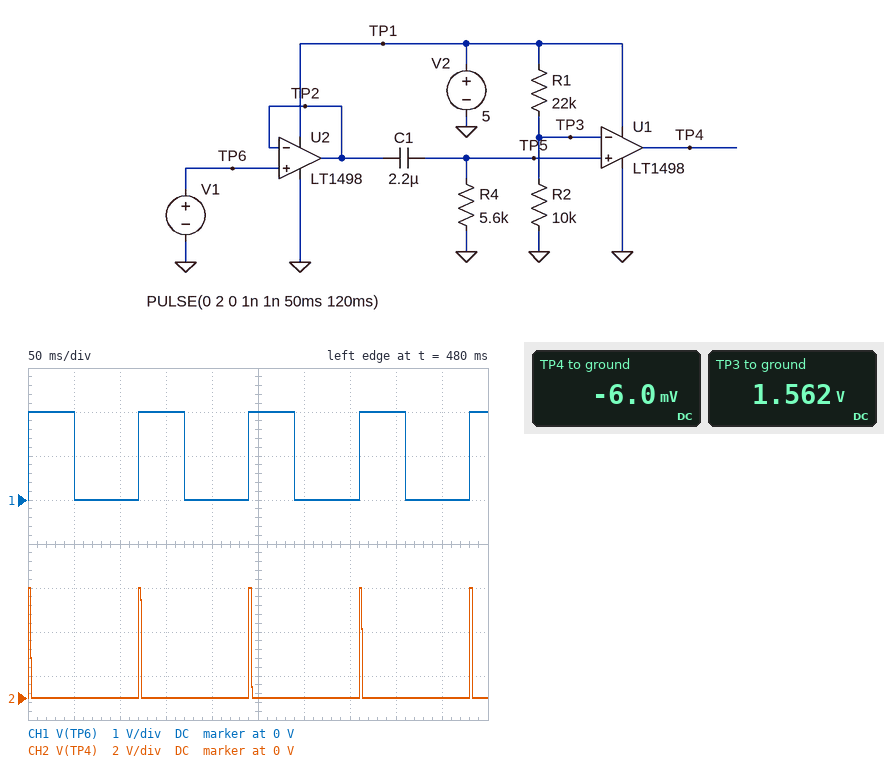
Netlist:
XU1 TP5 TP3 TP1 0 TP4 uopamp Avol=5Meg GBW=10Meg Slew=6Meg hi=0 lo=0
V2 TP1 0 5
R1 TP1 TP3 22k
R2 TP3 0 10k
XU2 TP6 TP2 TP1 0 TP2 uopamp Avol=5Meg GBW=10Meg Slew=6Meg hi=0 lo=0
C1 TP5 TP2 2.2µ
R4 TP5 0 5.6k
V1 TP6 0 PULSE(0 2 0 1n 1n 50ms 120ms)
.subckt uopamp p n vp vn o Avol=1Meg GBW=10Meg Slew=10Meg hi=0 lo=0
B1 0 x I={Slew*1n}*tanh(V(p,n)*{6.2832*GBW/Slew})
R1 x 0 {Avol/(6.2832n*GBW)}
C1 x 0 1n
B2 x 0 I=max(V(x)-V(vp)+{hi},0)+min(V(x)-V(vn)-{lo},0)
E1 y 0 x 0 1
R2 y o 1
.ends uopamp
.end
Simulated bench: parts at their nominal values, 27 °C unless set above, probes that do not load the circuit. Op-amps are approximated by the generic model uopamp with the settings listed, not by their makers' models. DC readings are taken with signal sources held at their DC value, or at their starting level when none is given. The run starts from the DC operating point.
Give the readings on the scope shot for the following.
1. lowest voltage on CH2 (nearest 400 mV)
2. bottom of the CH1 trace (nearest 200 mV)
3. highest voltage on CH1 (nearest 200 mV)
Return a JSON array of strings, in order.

["0 V", "0 V", "2.0 V"]
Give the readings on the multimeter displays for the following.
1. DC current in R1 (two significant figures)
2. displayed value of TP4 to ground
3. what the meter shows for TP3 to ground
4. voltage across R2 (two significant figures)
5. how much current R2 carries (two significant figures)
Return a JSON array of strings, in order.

["160 µA", "-6.0 mV", "1.562 V", "1.6 V", "160 µA"]
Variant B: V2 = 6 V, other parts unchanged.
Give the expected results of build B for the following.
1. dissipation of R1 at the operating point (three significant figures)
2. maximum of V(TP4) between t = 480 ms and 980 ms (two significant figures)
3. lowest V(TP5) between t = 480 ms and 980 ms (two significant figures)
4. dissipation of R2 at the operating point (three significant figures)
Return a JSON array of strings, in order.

["773 µW", "6.0 V", "-2.0 V", "352 µW"]
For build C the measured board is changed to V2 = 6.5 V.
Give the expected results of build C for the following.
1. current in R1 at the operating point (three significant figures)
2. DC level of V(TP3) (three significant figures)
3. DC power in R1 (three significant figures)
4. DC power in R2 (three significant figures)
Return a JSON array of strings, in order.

["203 µA", "2.03 V", "908 µW", "413 µW"]
